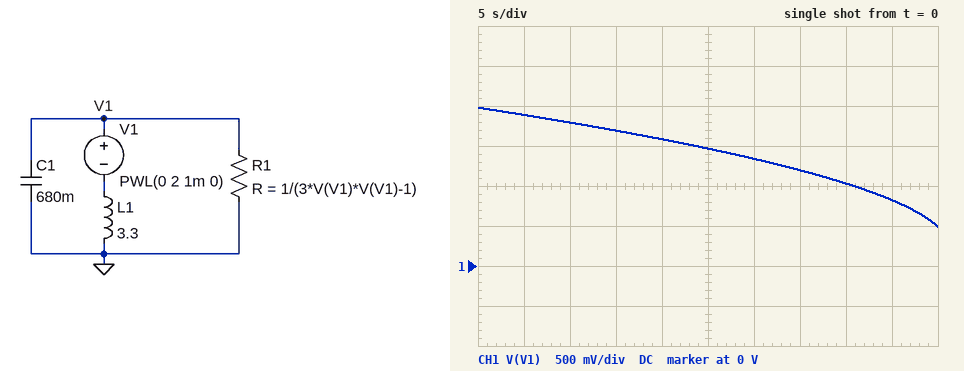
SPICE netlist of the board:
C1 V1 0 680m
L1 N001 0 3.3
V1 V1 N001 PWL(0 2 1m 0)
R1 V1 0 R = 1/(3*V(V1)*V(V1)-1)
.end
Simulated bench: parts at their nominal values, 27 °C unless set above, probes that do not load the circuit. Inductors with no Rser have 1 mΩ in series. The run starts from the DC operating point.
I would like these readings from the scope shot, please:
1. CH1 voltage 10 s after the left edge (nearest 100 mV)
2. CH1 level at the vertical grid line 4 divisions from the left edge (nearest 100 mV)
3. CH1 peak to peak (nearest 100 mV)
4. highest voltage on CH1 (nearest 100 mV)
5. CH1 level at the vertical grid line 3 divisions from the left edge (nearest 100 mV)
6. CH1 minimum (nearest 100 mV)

1.8 V
1.6 V
1.5 V
2.0 V
1.7 V
500 mV
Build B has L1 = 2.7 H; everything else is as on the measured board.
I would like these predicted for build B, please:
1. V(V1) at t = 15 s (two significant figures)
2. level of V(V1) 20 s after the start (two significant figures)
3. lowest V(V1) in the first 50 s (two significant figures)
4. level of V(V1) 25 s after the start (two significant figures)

1.6 V
1.5 V
-670 mV
1.3 V
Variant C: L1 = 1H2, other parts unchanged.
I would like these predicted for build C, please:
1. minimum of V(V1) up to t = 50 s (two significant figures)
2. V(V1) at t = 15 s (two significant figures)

-670 mV
990 mV
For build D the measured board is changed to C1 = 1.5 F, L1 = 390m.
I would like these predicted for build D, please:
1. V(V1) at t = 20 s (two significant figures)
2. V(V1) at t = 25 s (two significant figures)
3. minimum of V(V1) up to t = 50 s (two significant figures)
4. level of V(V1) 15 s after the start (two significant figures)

660 mV
670 mV
-690 mV
630 mV
